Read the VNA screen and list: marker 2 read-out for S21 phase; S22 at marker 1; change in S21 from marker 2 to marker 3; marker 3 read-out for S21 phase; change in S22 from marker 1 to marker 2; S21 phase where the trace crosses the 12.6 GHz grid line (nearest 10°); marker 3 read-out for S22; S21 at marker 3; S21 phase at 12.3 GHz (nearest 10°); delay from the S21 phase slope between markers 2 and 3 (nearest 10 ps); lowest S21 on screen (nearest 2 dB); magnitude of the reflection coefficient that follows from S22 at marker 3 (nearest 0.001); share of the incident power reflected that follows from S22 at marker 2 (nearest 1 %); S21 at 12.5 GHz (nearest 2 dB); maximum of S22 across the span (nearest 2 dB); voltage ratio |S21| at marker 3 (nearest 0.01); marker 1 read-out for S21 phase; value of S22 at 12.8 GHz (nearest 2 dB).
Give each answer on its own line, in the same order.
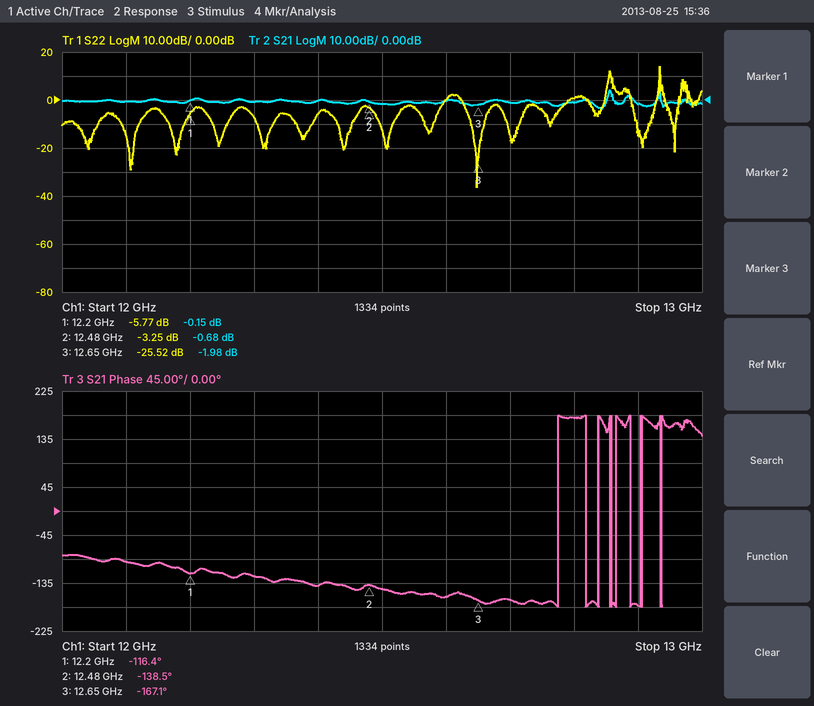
-138.5°
-5.77 dB
-1.30 dB
-167.1°
2.52 dB
-160°
-25.52 dB
-1.98 dB
-120°
470 ps
-4 dB
0.053
47 %
-2 dB
14 dB
0.80
-116.4°
0 dB
